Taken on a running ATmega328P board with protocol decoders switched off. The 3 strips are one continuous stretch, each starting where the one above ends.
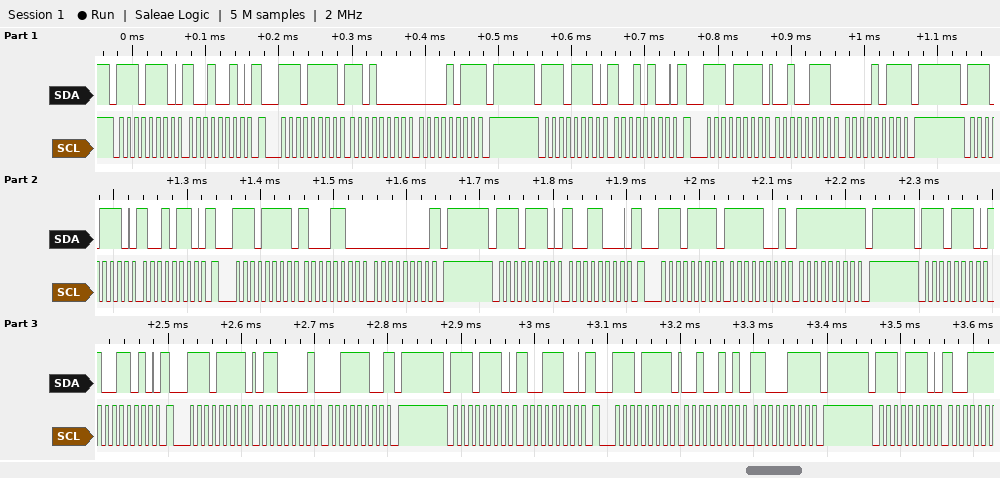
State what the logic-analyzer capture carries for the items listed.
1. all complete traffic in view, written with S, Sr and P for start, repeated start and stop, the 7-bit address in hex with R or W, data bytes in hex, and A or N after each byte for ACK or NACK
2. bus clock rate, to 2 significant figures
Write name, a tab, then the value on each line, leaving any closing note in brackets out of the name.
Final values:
all complete traffic in view, written with S, Sr and P for start, repeated start and stop, the 7-bit address in hex with R or W, data bytes in hex, and A or N after each byte for ACK or NACK	S 77W A 92 A Sr 77R A D0 A 0B N P S 77W A 94 A Sr 77R A 27 A 0B N P S 77W A 96 A Sr 77R A 8C A 00 N P S 77W A 98 A Sr 77R A F9 A FF N P S 77W A 9A A Sr 77R A 61 A 3C N P S 77W A 9C A Sr 77R A 25 A C7 N P S 77W A
bus clock rate, to 2 significant figures	100 kHz
